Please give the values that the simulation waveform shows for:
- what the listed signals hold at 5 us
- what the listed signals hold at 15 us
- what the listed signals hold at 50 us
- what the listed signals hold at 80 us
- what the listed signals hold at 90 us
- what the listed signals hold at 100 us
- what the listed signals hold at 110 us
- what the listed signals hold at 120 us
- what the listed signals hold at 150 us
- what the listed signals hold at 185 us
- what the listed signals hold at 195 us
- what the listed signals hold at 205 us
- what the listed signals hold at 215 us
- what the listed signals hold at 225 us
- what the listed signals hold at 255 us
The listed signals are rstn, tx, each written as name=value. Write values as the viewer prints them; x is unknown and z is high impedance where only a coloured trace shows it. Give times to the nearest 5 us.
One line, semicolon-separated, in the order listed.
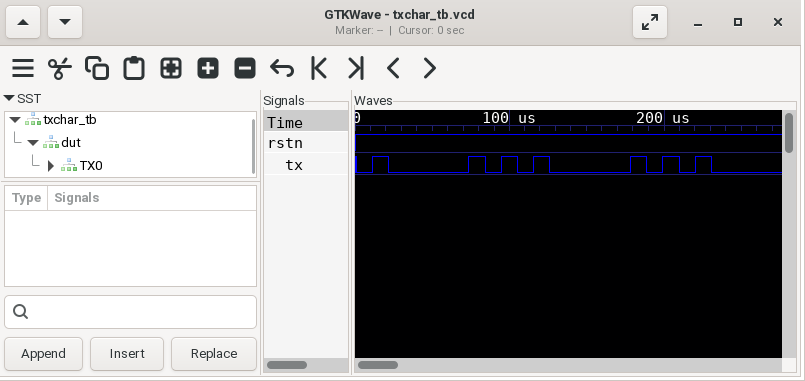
rstn=1, tx=0; rstn=1, tx=1; rstn=1, tx=0; rstn=1, tx=1; rstn=1, tx=0; rstn=1, tx=1; rstn=1, tx=0; rstn=1, tx=1; rstn=1, tx=0; rstn=1, tx=1; rstn=1, tx=0; rstn=1, tx=1; rstn=1, tx=0; rstn=1, tx=1; rstn=1, tx=0
